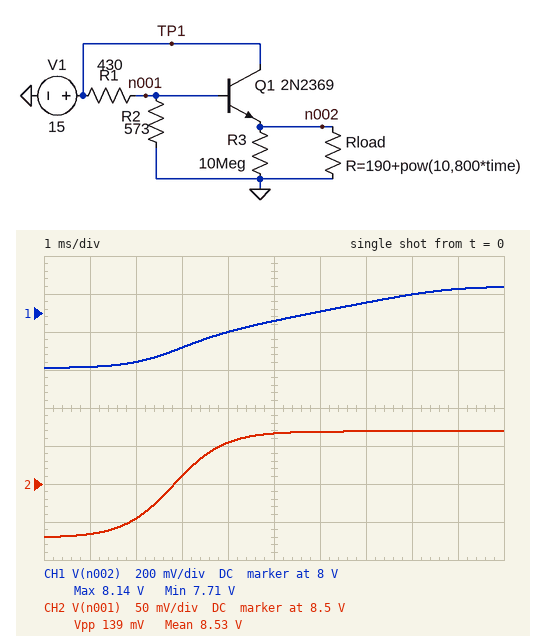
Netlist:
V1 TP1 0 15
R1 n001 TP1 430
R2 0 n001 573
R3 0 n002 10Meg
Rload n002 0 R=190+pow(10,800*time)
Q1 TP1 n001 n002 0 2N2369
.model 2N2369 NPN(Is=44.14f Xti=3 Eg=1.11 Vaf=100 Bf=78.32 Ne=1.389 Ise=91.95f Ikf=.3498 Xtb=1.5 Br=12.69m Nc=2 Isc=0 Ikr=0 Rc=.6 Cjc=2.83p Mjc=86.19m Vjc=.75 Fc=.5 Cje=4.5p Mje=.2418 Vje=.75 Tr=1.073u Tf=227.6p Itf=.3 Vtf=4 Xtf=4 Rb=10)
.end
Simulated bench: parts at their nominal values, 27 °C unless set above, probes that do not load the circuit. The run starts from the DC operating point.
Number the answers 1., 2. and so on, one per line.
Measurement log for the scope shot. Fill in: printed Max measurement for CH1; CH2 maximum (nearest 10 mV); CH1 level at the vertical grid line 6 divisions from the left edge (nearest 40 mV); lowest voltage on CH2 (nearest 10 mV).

1. 8.14 V
2. 8.57 V
3. 8.00 V
4. 8.43 V
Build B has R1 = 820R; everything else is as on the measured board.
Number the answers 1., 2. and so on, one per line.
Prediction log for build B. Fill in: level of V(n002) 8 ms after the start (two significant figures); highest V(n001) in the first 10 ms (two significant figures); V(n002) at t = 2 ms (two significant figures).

1. 5.7 V
2. 6.2 V
3. 5.4 V
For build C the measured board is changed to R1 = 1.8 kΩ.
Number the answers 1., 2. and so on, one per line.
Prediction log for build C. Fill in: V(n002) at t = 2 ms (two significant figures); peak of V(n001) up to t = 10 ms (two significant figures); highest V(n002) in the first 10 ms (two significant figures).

1. 2.9 V
2. 3.6 V
3. 3.2 V
